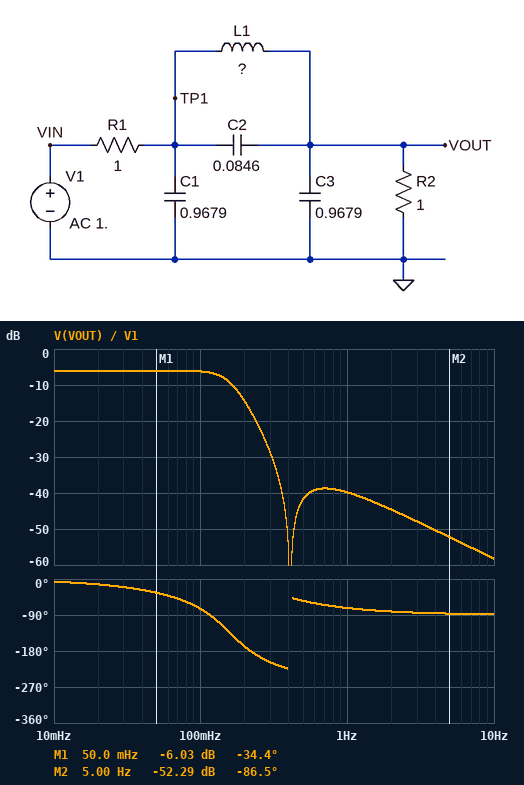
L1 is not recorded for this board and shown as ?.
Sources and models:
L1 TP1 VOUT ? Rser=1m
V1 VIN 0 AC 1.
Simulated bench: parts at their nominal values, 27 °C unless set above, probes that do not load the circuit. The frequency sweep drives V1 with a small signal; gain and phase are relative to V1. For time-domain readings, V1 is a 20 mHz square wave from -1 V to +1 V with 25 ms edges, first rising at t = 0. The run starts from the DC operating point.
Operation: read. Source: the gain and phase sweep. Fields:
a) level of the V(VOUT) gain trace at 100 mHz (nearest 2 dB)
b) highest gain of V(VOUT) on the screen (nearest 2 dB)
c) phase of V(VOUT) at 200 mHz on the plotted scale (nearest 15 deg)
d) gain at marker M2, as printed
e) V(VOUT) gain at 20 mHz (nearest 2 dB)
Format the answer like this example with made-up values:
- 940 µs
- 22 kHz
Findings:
- -6 dB
- -6 dB
- -165 deg
- -52.29 dB
- -6 dB
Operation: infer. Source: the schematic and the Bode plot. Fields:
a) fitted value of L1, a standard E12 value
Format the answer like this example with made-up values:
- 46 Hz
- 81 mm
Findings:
- 1.8 H
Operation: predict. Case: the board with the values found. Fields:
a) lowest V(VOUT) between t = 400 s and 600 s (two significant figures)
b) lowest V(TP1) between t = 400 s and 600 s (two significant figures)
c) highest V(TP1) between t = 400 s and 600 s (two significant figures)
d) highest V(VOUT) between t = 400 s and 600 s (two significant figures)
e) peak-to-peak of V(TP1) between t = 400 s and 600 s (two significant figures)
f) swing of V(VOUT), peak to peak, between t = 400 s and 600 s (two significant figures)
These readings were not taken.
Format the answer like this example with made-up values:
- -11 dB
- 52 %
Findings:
- -600 mV
- -800 mV
- 800 mV
- 600 mV
- 1.6 V
- 1.2 V
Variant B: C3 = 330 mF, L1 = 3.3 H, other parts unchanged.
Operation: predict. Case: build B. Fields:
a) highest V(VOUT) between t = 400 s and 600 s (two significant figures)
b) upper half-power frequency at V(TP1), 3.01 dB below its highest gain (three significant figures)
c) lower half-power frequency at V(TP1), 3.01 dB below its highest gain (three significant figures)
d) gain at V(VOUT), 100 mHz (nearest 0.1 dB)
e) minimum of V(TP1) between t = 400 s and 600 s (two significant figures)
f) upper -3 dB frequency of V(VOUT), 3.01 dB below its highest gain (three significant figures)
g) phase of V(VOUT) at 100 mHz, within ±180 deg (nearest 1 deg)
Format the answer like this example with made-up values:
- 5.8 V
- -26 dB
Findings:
- 530 mV
- 233 mHz
- 38.4 mHz
- -9.1 dB
- -970 mV
- 99.0 mHz
- -88 deg
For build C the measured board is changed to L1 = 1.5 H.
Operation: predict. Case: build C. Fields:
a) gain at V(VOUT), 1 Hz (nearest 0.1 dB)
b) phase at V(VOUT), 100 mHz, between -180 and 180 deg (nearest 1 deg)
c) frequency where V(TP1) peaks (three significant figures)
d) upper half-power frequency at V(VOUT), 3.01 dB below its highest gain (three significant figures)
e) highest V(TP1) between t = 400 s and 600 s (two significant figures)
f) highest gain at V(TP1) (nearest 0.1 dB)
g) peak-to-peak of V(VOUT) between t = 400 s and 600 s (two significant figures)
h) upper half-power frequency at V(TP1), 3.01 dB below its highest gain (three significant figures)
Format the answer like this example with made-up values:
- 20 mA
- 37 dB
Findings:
- -40.1 dB
- -67 deg
- 179 mHz
- 174 mHz
- 750 mV
- -2.1 dB
- 1.2 V
- 286 mHz
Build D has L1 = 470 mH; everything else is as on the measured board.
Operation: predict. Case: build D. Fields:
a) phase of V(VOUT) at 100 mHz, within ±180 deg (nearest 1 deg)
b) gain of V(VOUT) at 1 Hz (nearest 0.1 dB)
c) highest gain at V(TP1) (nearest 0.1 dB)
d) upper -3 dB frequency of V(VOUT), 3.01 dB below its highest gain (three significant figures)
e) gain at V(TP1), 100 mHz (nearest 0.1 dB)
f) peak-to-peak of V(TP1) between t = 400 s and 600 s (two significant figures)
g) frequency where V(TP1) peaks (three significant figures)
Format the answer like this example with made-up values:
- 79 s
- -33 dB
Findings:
- -41 deg
- -46.4 dB
- -3.7 dB
- 332 mHz
- -7.9 dB
- 1.1 V
- 321 mHz
